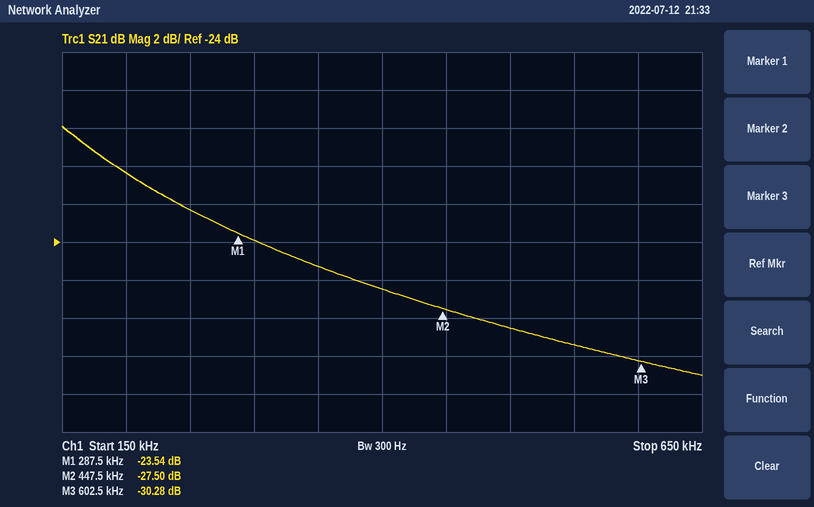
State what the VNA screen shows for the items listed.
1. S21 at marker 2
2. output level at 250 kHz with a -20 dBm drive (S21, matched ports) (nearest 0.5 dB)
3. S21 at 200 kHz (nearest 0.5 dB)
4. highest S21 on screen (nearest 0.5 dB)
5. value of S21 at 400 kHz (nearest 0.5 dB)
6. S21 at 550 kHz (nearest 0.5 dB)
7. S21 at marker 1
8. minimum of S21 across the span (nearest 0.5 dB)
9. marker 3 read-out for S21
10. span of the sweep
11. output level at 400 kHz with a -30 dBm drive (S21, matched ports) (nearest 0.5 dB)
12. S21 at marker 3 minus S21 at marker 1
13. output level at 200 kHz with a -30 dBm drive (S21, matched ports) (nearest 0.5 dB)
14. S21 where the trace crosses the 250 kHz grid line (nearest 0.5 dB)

-27.50 dB
-42.5 dBm
-20.5 dB
-18.0 dB
-26.5 dB
-29.5 dB
-23.54 dB
-31.0 dB
-30.28 dB
500 kHz
-56.5 dBm
-6.74 dB
-50.5 dBm
-22.5 dB
